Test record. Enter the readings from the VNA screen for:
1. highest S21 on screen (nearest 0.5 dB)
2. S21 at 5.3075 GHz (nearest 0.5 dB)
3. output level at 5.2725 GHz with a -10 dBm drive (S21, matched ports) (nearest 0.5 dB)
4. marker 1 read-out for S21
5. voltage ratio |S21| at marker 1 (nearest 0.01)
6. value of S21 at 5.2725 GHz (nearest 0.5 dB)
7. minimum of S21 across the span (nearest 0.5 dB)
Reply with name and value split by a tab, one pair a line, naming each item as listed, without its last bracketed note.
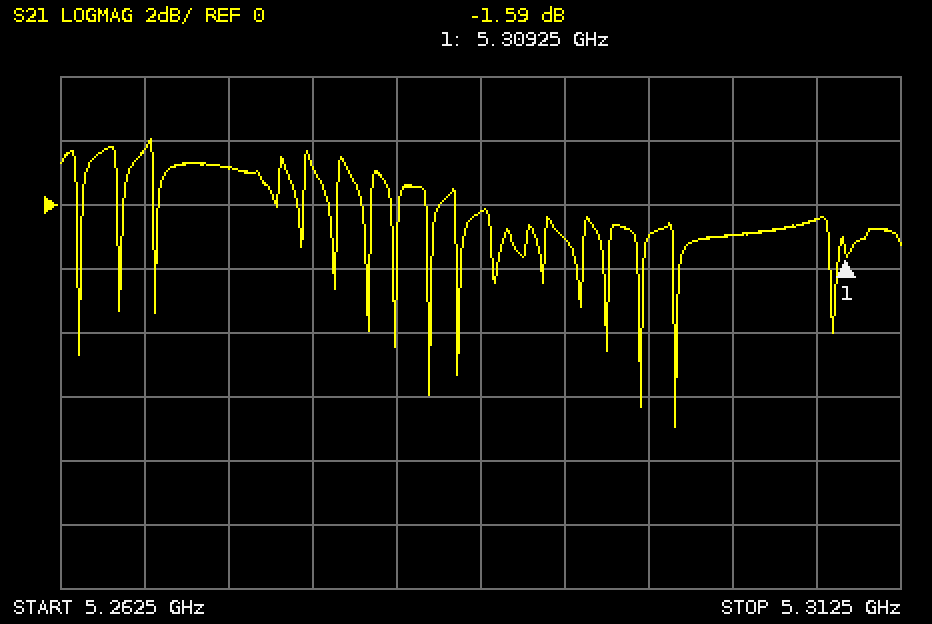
highest S21 on screen	2.0 dB
S21 at 5.3075 GHz	-0.5 dB
output level at 5.2725 GHz with a -10 dBm drive (S21, matched ports)	-9.0 dBm
marker 1 read-out for S21	-1.59 dB
voltage ratio |S21| at marker 1	0.83
value of S21 at 5.2725 GHz	1.0 dB
minimum of S21 across the span	-7.0 dB
